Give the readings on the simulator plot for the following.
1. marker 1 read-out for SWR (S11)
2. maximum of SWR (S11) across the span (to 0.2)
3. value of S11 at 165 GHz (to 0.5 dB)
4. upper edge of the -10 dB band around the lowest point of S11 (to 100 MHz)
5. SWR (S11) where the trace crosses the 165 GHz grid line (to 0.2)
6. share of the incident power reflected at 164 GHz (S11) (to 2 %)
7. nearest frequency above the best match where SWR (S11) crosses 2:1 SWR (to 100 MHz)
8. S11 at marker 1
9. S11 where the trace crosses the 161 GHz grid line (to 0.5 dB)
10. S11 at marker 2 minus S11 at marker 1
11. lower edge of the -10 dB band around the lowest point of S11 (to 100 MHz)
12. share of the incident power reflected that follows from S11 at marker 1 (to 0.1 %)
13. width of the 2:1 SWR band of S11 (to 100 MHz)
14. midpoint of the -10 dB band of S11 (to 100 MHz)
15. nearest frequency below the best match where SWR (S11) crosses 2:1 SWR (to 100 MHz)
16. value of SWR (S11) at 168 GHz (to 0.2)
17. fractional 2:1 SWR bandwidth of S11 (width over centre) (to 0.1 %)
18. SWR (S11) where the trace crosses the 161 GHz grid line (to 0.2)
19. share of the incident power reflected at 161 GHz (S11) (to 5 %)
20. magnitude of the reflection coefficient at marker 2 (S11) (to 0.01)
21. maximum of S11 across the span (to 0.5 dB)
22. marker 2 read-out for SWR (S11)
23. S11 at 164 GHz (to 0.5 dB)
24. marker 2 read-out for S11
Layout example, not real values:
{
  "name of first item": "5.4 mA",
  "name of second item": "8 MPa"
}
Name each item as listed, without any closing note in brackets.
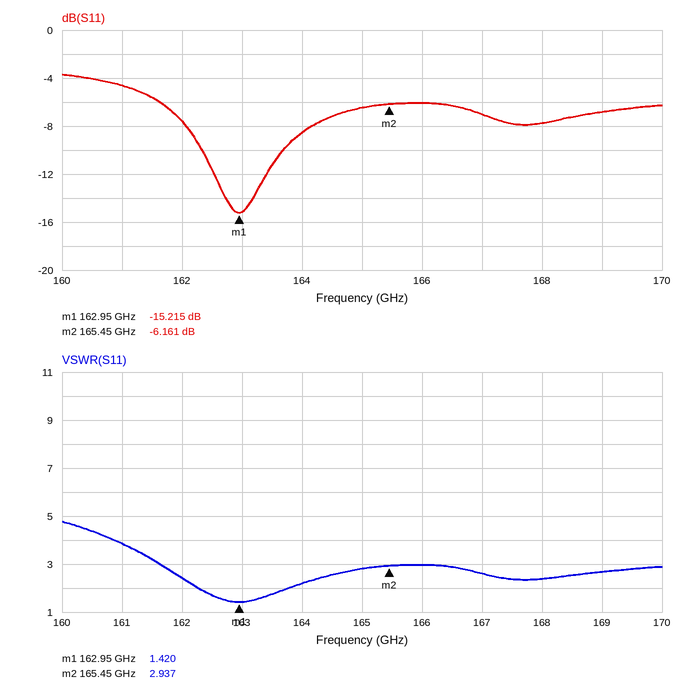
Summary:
{
  "marker 1 read-out for SWR": "1.420",
  "maximum of SWR (S11) across the span": "4.8",
  "value of S11 at 165 GHz": "-6.5 dB",
  "upper edge of the -10 dB band around the lowest point of S11": "163.7 GHz",
  "SWR (S11) where the trace crosses the 165 GHz grid line": "2.8",
  "share of the incident power reflected at 164 GHz (S11)": "14 %",
  "nearest frequency above the best match where SWR (S11) crosses 2:1 SWR": "163.8 GHz",
  "S11 at marker 1": "-15.215 dB",
  "S11 where the trace crosses the 161 GHz grid line": "-4.5 dB",
  "S11 at marker 2 minus S11 at marker 1": "9.054 dB",
  "lower edge of the -10 dB band around the lowest point of S11": "162.3 GHz",
  "share of the incident power reflected that follows from S11 at marker 1": "3.0 %",
  "width of the 2:1 SWR band of S11": "1.5 GHz",
  "midpoint of the -10 dB band of S11": "163.0 GHz",
  "nearest frequency below the best match where SWR (S11) crosses 2:1 SWR": "162.3 GHz",
  "value of SWR (S11) at 168 GHz": "2.4",
  "fractional 2:1 SWR bandwidth of S11 (width over centre)": "0.9 %",
  "SWR (S11) where the trace crosses the 161 GHz grid line": "3.8",
  "share of the incident power reflected at 161 GHz (S11)": "35 %",
  "magnitude of the reflection coefficient at marker 2 (S11)": "0.49",
  "maximum of S11 across the span": "-3.5 dB",
  "marker 2 read-out for SWR": "2.937",
  "S11 at 164 GHz": "-8.5 dB",
  "marker 2 read-out for S11": "-6.161 dB"
}
